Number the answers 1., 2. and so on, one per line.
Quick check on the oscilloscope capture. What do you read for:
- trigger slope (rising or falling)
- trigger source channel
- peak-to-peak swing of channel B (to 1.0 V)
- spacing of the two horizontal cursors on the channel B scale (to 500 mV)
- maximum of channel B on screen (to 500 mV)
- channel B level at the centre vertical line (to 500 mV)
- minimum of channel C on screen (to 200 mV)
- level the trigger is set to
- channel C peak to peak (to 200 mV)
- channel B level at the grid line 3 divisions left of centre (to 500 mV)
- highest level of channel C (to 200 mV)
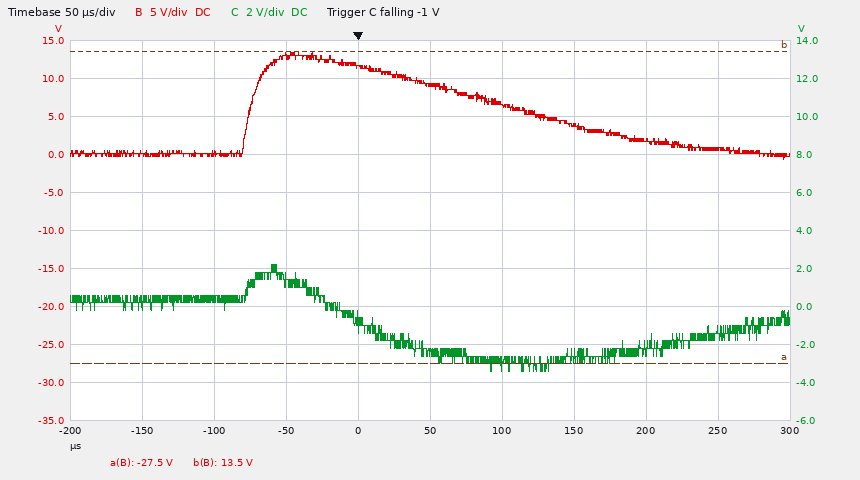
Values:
1. falling
2. channel C
3. 14.0 V
4. 41.0 V
5. 13.5 V
6. 9.0 V
7. -3.4 V
8. -1 V
9. 5.6 V
10. 0.0 V
11. 2.2 V
